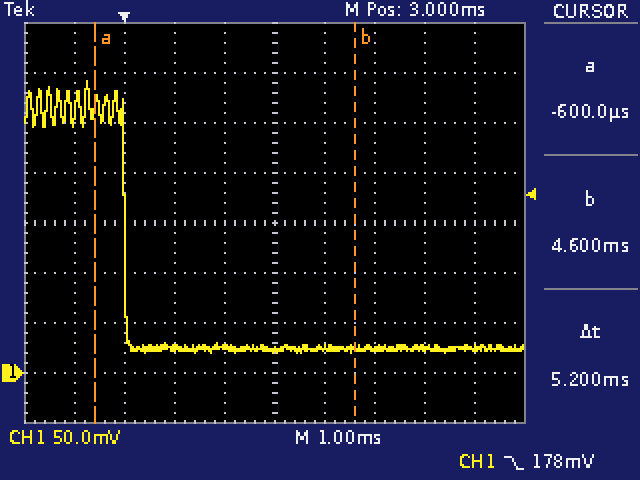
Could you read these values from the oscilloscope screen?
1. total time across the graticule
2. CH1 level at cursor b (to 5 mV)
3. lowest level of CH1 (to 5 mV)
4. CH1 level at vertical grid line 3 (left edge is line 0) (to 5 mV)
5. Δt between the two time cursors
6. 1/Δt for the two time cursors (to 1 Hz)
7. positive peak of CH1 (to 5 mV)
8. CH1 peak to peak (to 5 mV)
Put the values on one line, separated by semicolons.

10 ms; 25 mV; 20 mV; 25 mV; 5.2 ms; 192 Hz; 290 mV; 270 mV
